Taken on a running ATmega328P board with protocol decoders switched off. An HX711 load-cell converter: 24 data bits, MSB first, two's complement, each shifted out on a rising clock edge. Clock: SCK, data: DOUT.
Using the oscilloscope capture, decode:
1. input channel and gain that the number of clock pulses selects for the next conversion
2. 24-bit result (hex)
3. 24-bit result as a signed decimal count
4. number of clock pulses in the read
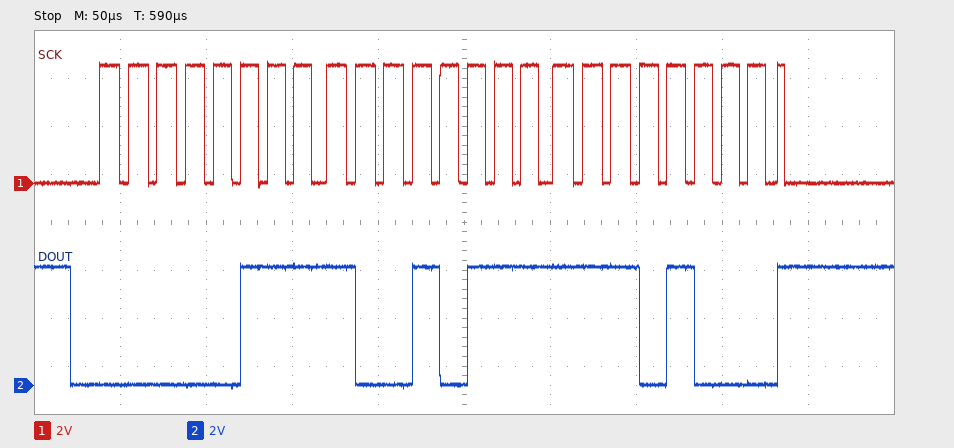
channel A, gain 128
0x0797E8
497640
25
